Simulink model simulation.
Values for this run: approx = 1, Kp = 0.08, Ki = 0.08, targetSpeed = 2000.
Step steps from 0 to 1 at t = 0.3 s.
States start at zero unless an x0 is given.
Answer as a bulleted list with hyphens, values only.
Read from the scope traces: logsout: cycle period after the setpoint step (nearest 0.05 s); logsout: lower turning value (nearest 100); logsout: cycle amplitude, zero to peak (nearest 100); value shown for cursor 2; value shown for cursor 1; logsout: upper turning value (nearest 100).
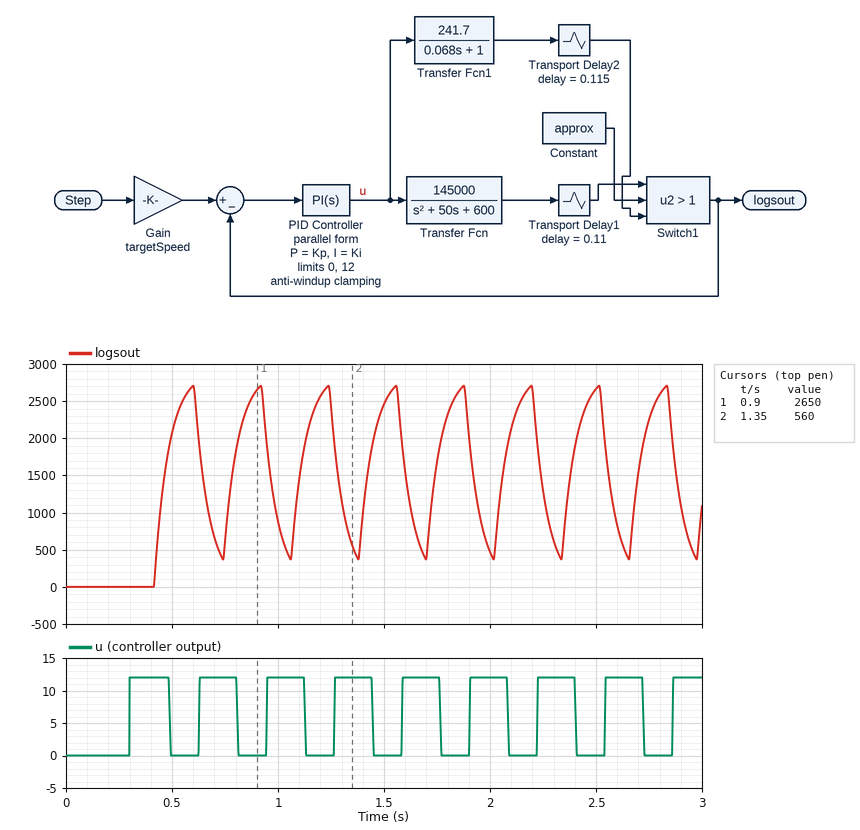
- 0.30 s
- 400
- 1200
- 560
- 2650
- 2700
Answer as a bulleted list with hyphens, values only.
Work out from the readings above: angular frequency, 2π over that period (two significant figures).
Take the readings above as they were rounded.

- 21 rad/s
